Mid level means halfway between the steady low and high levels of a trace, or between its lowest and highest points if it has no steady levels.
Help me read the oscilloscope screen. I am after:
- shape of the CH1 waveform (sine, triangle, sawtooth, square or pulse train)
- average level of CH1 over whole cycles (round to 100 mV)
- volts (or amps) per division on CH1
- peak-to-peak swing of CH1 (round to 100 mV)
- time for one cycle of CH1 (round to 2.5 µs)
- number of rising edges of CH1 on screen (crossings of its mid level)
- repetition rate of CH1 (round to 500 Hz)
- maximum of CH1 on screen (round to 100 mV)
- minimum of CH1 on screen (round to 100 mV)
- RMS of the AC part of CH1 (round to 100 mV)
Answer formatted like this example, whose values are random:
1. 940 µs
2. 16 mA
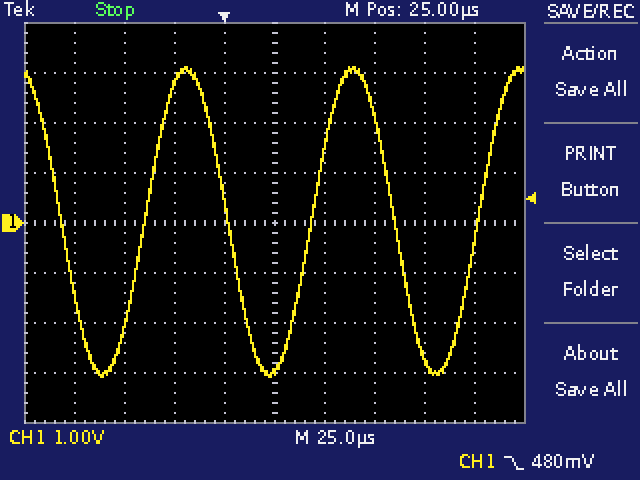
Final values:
1. sine
2. 0.0 V
3. 1 V
4. 6.2 V
5. 82.5 µs
6. 3
7. 12.0 kHz
8. 3.1 V
9. -3.1 V
10. 2.2 V
